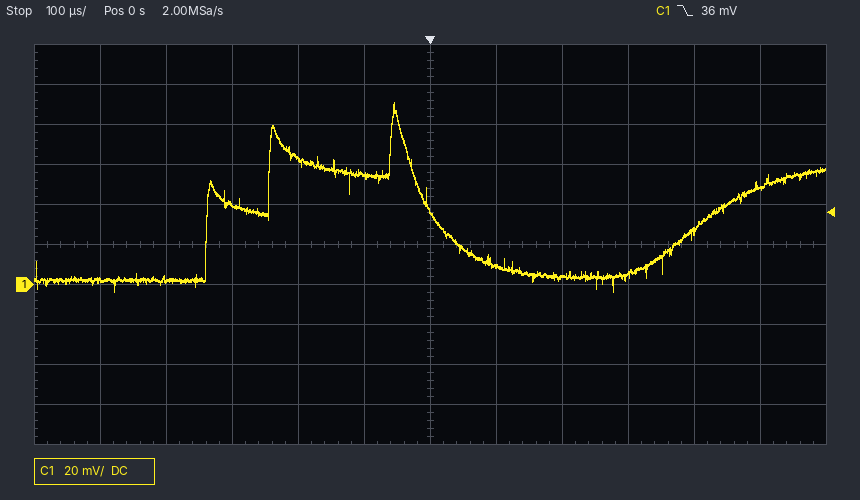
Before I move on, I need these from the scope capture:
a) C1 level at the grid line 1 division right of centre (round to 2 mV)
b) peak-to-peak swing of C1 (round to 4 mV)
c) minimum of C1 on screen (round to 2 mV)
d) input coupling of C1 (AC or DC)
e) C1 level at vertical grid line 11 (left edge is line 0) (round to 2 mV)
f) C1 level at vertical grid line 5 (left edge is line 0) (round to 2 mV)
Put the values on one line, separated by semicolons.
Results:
10 mV; 96 mV; -4 mV; DC; 48 mV; 54 mV
